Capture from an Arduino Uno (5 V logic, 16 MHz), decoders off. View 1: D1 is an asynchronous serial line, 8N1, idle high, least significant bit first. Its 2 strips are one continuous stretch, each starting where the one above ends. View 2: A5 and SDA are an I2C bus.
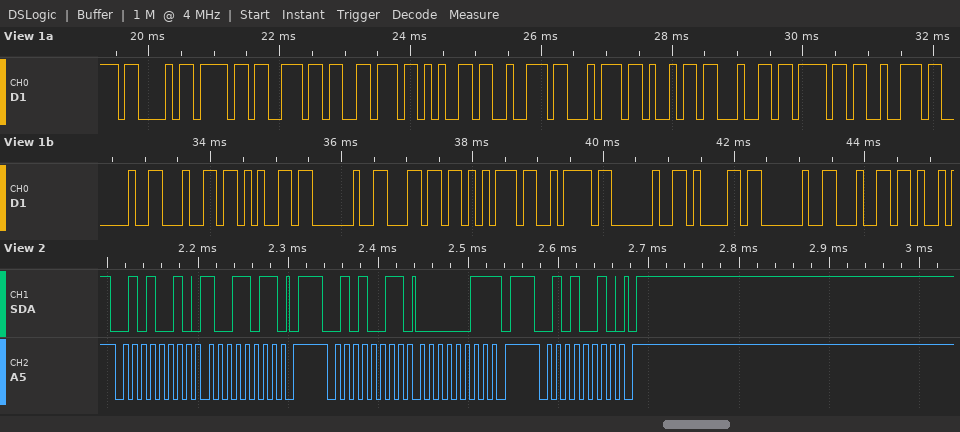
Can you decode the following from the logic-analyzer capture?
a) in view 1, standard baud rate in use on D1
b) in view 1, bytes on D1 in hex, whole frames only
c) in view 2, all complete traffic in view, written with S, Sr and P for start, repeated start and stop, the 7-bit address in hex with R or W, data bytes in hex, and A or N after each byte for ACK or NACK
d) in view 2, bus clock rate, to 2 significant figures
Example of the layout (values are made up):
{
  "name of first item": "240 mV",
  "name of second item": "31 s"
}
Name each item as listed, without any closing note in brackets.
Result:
{
  "in view 1, standard baud rate in use on D1": "9600 baud",
  "in view 1, bytes on D1 in hex, whole frames only": "0x43 0x6F 0x6E 0x76 0x65 0x72 0x74 0x69 0x64 0x6F 0x72 0x20 0x64 0x65 0x20 0x6C 0x75 0x7A 0x20 0x61 0x20 0x64",
  "in view 2, all complete traffic in view, written with S, Sr and P for start, repeated start and stop, the 7-bit address in hex with R or W, data bytes in hex, and A or N after each byte for ACK or NACK": "S 29W A 9B A P S 29R A 03 N P S 29W A P",
  "in view 2, bus clock rate, to 2 significant figures": "100 kHz"
}
